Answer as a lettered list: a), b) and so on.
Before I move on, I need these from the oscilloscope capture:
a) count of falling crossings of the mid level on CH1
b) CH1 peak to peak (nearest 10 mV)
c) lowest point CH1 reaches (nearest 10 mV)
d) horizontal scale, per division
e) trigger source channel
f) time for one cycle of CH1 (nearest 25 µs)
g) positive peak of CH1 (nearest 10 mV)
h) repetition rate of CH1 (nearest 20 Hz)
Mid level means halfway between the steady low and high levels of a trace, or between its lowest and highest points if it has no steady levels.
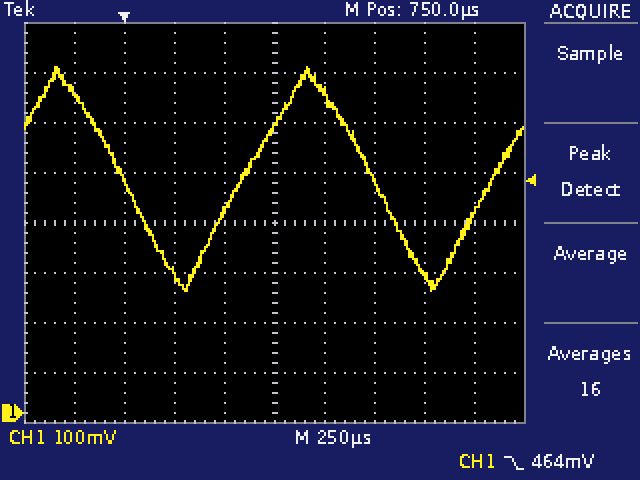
a) 2
b) 450 mV
c) 240 mV
d) 250 µs
e) CH1
f) 1.250 ms
g) 690 mV
h) 800 Hz
